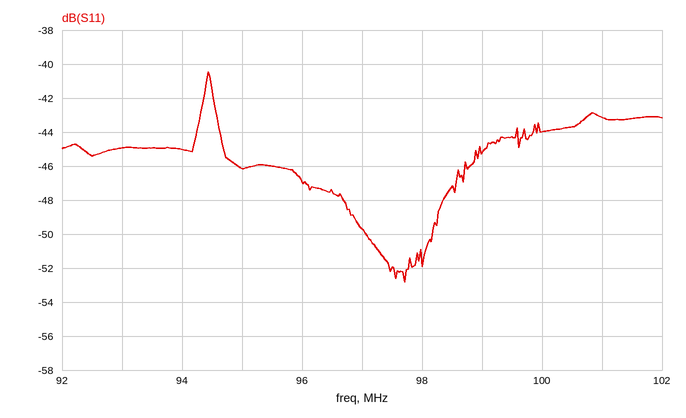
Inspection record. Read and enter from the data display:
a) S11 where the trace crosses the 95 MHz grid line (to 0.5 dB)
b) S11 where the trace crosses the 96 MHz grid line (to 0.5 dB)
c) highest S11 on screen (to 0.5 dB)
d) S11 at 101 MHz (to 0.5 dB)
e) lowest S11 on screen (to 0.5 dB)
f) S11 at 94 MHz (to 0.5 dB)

-46.0 dB
-47.0 dB
-40.5 dB
-43.0 dB
-53.0 dB
-45.0 dB
